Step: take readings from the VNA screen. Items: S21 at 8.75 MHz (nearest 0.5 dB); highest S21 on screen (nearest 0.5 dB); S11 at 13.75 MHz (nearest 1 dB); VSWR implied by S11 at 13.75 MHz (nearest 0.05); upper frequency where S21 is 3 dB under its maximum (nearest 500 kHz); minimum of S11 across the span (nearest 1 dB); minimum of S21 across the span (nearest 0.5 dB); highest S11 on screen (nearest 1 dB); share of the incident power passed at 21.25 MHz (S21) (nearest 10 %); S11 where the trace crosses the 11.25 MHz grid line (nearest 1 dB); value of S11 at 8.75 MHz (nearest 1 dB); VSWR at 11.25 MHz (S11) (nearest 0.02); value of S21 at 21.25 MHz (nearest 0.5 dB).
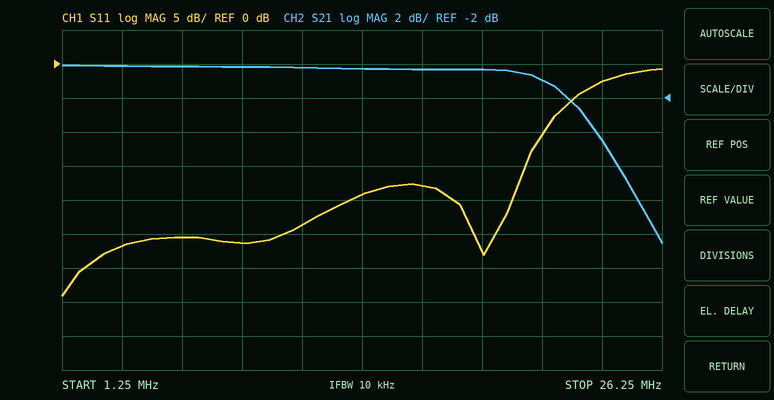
0.0 dB
0.0 dB
-19 dB
1.25
23.0 MHz
-34 dB
-10.5 dB
-1 dB
80 %
-24 dB
-26 dB
1.14
-1.0 dB
